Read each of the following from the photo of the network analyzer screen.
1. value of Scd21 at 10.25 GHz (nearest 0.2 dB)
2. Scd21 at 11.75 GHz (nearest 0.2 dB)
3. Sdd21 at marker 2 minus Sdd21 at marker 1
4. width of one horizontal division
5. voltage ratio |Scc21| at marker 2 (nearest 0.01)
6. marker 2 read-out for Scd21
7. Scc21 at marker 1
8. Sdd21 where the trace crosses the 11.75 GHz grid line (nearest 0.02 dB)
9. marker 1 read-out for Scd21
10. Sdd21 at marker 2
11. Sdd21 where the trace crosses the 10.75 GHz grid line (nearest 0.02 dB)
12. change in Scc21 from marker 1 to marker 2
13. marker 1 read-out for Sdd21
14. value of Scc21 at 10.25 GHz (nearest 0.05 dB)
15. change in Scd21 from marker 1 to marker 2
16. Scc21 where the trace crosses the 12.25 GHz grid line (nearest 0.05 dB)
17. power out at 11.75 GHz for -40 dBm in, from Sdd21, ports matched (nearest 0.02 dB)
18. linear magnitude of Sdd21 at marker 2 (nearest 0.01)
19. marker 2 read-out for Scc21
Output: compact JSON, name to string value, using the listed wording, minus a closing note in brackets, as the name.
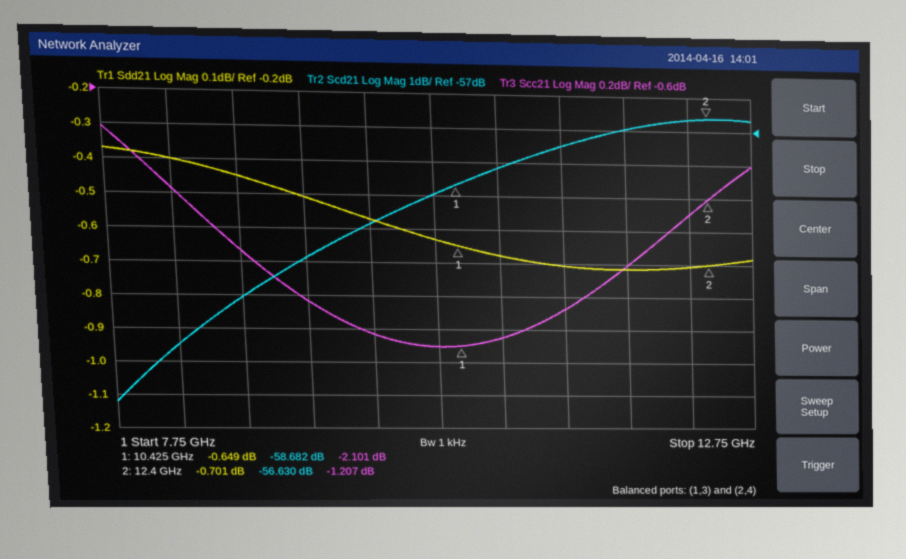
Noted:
{"value of Scd21 at 10.25 GHz": "-59.0 dB", "Scd21 at 11.75 GHz": "-57.0 dB", "Sdd21 at marker 2 minus Sdd21 at marker 1": "-0.052 dB", "width of one horizontal division": "500 MHz", "voltage ratio |Scc21| at marker 2": "0.87", "marker 2 read-out for Scd21": "-56.630 dB", "Scc21 at marker 1": "-2.101 dB", "Sdd21 where the trace crosses the 11.75 GHz grid line": "-0.72 dB", "marker 1 read-out for Scd21": "-58.682 dB", "Sdd21 at marker 2": "-0.701 dB", "Sdd21 where the trace crosses the 10.75 GHz grid line": "-0.68 dB", "change in Scc21 from marker 1 to marker 2": "0.894 dB", "marker 1 read-out for Sdd21": "-0.649 dB", "value of Scc21 at 10.25 GHz": "-2.10 dB", "change in Scd21 from marker 1 to marker 2": "2.052 dB", "Scc21 where the trace crosses the 12.25 GHz grid line": "-1.30 dB", "power out at 11.75 GHz for -40 dBm in, from Sdd21, ports matched": "-40.72 dBm", "linear magnitude of Sdd21 at marker 2": "0.92", "marker 2 read-out for Scc21": "-1.207 dB"}
